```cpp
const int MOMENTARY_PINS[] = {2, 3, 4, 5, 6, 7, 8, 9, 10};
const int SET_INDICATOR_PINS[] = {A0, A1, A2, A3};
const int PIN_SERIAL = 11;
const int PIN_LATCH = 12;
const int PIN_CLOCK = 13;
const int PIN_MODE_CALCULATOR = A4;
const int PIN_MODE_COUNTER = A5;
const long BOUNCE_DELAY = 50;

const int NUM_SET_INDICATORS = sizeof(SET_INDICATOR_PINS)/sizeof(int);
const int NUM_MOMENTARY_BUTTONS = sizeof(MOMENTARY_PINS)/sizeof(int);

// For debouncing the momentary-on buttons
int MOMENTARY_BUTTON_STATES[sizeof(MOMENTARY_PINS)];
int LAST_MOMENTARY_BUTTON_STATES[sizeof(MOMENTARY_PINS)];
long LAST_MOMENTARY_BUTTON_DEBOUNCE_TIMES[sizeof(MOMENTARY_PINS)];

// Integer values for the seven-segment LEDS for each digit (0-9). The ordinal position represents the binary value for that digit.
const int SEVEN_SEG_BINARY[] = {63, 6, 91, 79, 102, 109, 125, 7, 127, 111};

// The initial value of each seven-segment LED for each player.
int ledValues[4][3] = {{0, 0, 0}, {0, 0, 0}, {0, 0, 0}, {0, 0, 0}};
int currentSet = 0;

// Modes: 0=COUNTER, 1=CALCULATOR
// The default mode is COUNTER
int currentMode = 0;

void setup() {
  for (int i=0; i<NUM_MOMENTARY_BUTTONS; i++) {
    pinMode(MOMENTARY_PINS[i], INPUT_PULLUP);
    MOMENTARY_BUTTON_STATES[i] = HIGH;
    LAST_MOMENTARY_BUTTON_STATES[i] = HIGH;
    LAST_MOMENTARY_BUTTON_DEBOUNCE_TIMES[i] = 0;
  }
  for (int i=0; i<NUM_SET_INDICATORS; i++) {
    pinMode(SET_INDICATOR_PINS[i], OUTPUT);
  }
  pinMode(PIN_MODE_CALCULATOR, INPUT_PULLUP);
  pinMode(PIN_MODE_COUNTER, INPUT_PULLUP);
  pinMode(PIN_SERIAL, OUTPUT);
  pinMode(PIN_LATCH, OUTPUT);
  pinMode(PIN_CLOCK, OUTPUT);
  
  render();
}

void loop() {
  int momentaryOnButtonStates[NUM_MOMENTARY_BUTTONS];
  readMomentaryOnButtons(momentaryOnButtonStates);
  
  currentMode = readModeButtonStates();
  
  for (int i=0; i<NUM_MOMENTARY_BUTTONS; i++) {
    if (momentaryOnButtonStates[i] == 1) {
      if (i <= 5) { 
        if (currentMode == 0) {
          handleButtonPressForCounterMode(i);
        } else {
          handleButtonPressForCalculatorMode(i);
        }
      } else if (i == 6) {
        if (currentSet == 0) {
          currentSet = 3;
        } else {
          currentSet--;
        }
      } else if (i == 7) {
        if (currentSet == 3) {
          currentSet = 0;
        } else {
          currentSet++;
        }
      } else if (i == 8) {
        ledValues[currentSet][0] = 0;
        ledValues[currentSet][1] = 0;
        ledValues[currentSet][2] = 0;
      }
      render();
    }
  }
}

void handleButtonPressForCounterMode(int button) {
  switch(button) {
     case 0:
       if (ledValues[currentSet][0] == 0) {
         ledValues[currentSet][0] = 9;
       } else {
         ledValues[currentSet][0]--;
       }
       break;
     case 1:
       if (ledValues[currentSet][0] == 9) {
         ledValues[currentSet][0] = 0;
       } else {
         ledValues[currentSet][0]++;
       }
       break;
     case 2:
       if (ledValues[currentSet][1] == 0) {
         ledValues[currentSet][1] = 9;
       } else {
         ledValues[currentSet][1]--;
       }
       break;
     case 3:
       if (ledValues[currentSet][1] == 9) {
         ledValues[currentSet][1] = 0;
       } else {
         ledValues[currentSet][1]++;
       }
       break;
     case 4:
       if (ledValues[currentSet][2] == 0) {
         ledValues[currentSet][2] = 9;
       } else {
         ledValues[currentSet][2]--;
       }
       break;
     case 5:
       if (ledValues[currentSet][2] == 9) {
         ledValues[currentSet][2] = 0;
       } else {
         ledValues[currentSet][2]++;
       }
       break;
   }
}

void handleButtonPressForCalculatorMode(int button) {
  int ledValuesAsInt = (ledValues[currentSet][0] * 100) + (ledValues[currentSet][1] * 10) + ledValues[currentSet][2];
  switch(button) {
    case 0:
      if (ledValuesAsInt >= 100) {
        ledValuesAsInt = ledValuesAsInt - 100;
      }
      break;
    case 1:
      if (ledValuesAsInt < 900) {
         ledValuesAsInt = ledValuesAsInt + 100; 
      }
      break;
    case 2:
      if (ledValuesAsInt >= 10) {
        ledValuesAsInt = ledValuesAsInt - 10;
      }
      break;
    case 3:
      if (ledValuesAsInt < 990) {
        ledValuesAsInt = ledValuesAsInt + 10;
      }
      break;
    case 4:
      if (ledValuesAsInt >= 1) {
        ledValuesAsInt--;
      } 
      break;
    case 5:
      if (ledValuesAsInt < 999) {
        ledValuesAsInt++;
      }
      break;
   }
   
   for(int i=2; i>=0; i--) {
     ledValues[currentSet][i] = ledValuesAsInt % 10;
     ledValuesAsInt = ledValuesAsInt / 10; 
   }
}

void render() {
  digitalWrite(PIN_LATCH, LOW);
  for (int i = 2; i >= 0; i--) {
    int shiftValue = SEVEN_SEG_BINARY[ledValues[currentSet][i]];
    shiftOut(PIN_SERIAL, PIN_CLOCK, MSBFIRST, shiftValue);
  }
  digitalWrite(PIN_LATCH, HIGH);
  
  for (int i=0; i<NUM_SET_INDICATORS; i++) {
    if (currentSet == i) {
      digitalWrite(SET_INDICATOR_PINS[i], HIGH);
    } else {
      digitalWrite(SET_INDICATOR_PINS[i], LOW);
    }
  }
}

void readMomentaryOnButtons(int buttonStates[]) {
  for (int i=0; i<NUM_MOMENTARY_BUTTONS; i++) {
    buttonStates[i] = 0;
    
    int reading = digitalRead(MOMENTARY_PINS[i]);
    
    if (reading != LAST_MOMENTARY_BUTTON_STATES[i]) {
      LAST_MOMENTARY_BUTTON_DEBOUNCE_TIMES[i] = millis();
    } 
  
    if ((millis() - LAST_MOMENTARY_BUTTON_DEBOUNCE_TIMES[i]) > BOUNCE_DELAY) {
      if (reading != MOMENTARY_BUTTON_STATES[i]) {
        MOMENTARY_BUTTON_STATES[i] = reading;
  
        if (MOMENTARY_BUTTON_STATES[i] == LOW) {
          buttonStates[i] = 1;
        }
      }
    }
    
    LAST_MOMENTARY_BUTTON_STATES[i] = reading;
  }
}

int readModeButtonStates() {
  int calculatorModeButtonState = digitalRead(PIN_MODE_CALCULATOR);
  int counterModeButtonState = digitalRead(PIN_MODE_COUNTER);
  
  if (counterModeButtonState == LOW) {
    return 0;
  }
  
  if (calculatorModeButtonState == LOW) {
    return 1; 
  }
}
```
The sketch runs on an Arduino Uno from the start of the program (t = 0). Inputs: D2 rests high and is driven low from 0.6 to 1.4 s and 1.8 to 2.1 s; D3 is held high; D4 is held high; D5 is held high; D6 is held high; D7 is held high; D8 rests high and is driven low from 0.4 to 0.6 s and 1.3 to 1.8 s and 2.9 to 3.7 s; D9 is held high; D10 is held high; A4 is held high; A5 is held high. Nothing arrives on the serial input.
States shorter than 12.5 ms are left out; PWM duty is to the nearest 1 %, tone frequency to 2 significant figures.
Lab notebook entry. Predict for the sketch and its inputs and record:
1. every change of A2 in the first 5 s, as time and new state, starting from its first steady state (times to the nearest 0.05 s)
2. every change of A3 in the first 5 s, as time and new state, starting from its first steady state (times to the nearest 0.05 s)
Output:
0 s low; 1.35 s high; 2.95 s low
0 s low; 0.45 s high; 1.35 s low
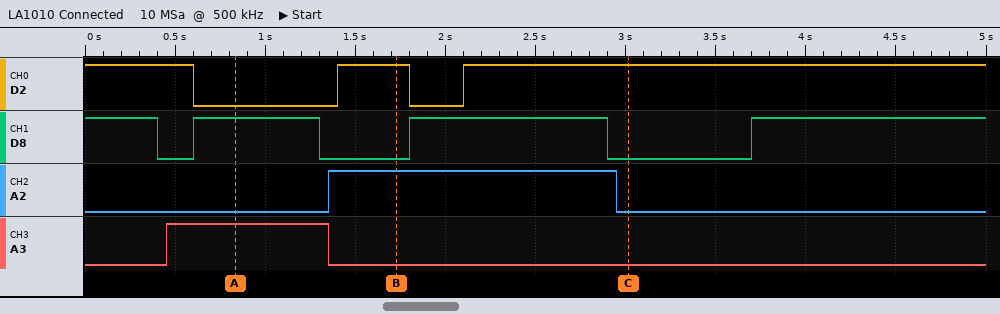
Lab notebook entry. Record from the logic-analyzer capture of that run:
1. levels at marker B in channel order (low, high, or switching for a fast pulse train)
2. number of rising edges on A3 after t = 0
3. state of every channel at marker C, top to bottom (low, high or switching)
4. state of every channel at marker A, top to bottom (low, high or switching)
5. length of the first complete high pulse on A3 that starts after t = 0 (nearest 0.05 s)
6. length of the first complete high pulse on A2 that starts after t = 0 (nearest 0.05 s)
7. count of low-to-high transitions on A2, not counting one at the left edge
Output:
D2 high, D8 low, A2 high, A3 low
1
D2 high, D8 low, A2 low, A3 low
D2 low, D8 high, A2 low, A3 high
0.90 s
1.60 s
1
